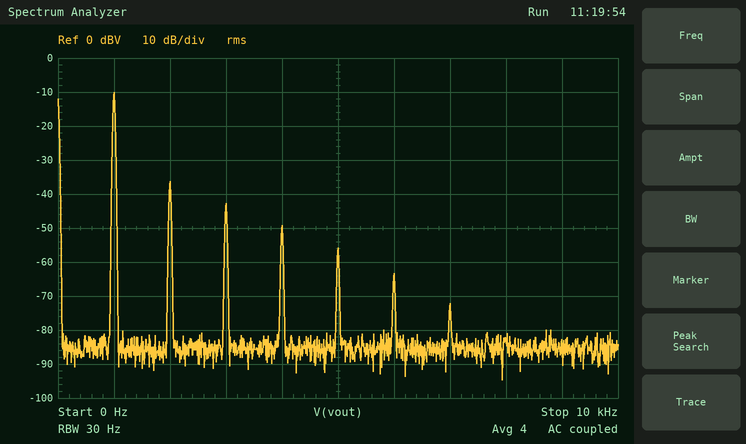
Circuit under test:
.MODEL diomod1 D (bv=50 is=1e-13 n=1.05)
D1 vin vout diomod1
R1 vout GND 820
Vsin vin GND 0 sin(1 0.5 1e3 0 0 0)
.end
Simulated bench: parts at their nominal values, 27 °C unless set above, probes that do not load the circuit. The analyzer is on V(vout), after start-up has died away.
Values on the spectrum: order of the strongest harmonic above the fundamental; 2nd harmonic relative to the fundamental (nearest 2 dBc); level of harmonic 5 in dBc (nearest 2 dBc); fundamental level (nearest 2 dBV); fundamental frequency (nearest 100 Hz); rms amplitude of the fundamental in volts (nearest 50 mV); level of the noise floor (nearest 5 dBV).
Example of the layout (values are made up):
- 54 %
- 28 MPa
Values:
- 2
- -26 dBc
- -46 dBc
- -10 dBV
- 1.0 kHz
- 300 mV
- -85 dBV
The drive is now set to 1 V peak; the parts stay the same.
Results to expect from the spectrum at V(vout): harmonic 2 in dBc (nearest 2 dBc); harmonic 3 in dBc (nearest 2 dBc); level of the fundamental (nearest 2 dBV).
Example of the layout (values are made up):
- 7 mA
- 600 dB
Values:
- -14 dBc
- -22 dBc
- -6 dBV
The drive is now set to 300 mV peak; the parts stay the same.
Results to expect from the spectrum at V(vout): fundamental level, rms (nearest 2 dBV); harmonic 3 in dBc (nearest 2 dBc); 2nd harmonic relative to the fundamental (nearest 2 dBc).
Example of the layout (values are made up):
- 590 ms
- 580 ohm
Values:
- -14 dBV
- -50 dBc
- -36 dBc
